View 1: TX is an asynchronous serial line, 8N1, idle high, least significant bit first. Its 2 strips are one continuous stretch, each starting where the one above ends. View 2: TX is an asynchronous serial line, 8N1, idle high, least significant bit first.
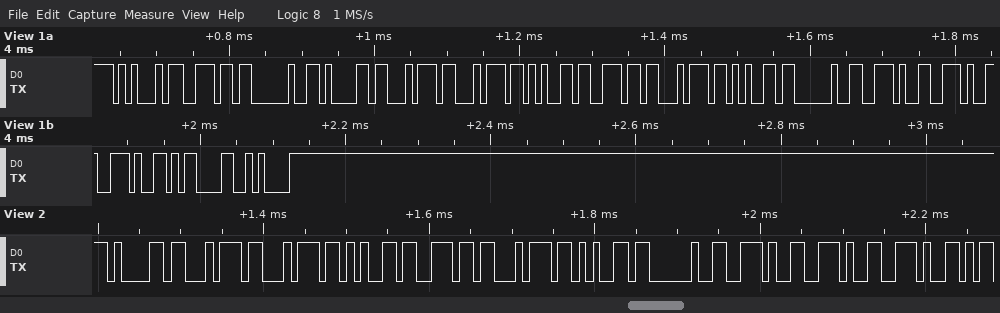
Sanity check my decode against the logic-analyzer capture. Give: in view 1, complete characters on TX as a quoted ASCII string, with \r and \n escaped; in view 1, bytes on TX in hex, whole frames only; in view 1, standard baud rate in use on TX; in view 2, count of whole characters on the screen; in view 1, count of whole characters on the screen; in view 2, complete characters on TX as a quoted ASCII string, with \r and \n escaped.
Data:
"En attente ...\r\n"
45 6E 20 61 74 74 65 6E 74 65 20 2E 2E 2E 0D 0A
115200 baud
11
16
"attente ..."
